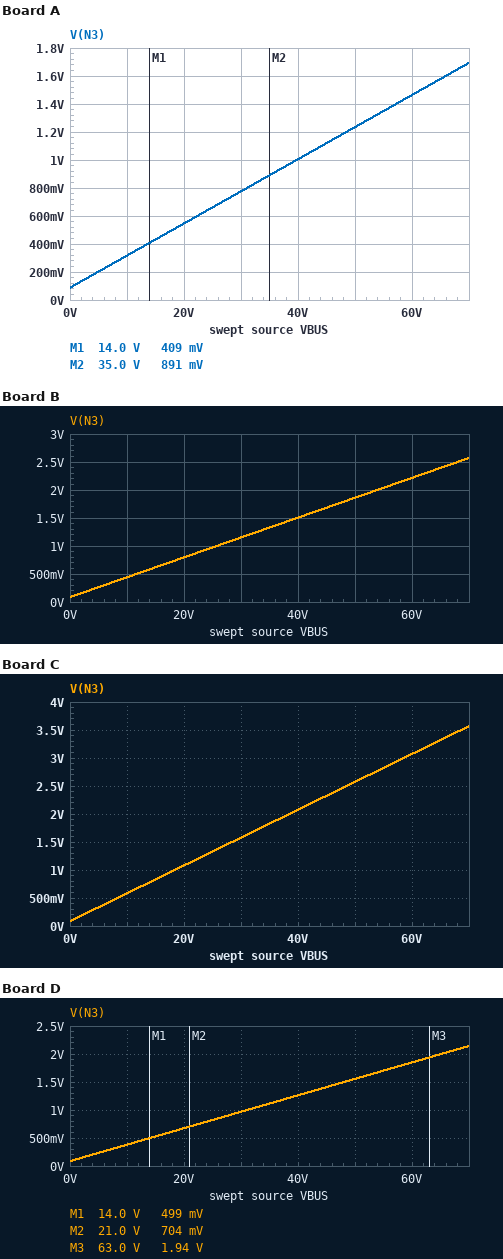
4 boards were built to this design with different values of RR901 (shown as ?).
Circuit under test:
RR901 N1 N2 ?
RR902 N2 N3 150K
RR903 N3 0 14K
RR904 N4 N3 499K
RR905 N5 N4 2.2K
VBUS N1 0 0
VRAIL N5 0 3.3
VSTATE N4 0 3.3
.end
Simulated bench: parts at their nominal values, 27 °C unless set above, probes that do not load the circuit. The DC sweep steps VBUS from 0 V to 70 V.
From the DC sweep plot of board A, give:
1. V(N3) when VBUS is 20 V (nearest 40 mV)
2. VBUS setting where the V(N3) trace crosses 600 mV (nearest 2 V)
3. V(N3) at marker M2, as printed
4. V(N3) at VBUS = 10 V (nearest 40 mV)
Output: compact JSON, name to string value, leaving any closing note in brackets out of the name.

{"V(N3) when VBUS is 20 V": "560 mV", "VBUS setting where the V(N3) trace crosses 600 mV": "22 V", "V(N3) at marker M2, as printed": "891 mV", "V(N3) at VBUS = 10 V": "320 mV"}
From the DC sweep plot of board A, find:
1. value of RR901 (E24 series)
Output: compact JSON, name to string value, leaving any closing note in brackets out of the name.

{"value of RR901": "430 kΩ"}
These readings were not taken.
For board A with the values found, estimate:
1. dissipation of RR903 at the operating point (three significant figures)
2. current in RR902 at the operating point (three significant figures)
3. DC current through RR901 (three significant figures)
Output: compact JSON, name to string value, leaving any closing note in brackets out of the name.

{"dissipation of RR903 at the operating point": "553 nW", "current in RR902 at the operating point": "152 nA", "DC current through RR901": "152 nA"}
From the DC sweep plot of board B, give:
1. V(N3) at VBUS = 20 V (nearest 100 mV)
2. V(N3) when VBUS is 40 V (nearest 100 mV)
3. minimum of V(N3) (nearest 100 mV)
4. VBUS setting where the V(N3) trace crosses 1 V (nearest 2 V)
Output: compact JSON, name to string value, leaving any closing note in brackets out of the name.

{"V(N3) at VBUS = 20 V": "800 mV", "V(N3) when VBUS is 40 V": "1.5 V", "minimum of V(N3)": "100 mV", "VBUS setting where the V(N3) trace crosses 1 V": "26 V"}
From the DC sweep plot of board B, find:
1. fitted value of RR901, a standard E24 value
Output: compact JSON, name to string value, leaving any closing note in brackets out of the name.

{"fitted value of RR901, a standard E24 value": "220 kΩ"}
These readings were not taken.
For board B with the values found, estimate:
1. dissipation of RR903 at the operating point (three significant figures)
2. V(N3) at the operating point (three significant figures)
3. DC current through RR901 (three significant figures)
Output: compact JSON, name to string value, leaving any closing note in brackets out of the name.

{"dissipation of RR903 at the operating point": "539 nW", "V(N3) at the operating point": "86.9 mV", "DC current through RR901": "235 nA"}
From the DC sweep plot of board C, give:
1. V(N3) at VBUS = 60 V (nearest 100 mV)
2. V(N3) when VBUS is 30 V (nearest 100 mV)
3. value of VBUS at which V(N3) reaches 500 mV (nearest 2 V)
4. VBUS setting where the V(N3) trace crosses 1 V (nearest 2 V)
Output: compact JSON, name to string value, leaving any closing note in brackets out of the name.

{"V(N3) at VBUS = 60 V": "3.1 V", "V(N3) when VBUS is 30 V": "1.6 V", "value of VBUS at which V(N3) reaches 500 mV": "8 V", "VBUS setting where the V(N3) trace crosses 1 V": "18 V"}
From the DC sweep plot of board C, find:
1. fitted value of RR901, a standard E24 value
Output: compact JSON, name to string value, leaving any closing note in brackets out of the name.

{"fitted value of RR901, a standard E24 value": "110 kΩ"}
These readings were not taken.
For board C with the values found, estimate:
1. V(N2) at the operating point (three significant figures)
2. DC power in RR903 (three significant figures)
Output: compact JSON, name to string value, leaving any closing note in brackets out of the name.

{"V(N2) at the operating point": "36.2 mV", "DC power in RR903": "523 nW"}
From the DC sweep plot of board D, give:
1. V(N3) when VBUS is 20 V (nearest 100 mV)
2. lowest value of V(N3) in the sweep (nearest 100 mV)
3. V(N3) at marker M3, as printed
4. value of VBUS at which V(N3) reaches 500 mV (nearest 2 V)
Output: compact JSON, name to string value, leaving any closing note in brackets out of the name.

{"V(N3) when VBUS is 20 V": "700 mV", "lowest value of V(N3) in the sweep": "100 mV", "V(N3) at marker M3, as printed": "1.94 V", "value of VBUS at which V(N3) reaches 500 mV": "14 V"}
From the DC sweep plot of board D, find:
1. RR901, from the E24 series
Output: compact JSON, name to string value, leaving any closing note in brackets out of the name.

{"RR901, from the E24 series": "300 kΩ"}
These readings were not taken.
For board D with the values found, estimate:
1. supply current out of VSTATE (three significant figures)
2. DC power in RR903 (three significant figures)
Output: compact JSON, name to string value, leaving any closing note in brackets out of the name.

{"supply current out of VSTATE": "6.44 µA", "DC power in RR903": "546 nW"}
